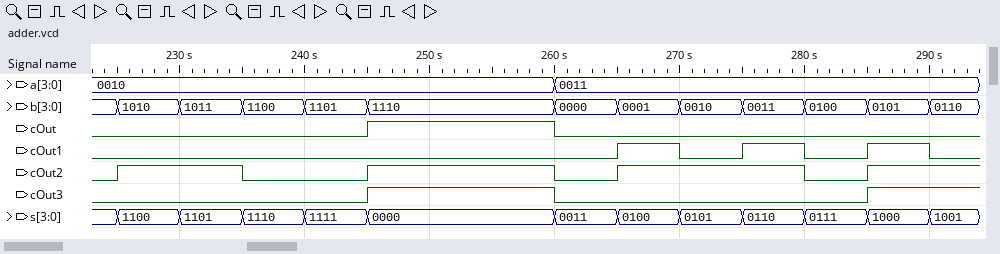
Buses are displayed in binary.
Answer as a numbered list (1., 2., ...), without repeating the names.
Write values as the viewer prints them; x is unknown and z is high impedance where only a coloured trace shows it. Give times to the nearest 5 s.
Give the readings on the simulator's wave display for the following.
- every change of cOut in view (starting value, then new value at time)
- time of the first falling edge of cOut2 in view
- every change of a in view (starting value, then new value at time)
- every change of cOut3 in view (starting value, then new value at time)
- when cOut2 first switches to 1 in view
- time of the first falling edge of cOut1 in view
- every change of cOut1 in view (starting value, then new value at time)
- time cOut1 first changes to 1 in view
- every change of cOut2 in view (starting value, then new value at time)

1. 0, 1 at 245 s, 0 at 260 s
2. 235 s
3. 0010, 0011 at 260 s
4. 0, 1 at 245 s, 0 at 260 s, 1 at 285 s
5. 225 s
6. 270 s
7. 0, 1 at 265 s, 0 at 270 s, 1 at 275 s, 0 at 280 s, 1 at 285 s, 0 at 290 s
8. 265 s
9. 0, 1 at 225 s, 0 at 235 s, 1 at 245 s, 0 at 260 s, 1 at 265 s, 0 at 280 s, 1 at 285 s
